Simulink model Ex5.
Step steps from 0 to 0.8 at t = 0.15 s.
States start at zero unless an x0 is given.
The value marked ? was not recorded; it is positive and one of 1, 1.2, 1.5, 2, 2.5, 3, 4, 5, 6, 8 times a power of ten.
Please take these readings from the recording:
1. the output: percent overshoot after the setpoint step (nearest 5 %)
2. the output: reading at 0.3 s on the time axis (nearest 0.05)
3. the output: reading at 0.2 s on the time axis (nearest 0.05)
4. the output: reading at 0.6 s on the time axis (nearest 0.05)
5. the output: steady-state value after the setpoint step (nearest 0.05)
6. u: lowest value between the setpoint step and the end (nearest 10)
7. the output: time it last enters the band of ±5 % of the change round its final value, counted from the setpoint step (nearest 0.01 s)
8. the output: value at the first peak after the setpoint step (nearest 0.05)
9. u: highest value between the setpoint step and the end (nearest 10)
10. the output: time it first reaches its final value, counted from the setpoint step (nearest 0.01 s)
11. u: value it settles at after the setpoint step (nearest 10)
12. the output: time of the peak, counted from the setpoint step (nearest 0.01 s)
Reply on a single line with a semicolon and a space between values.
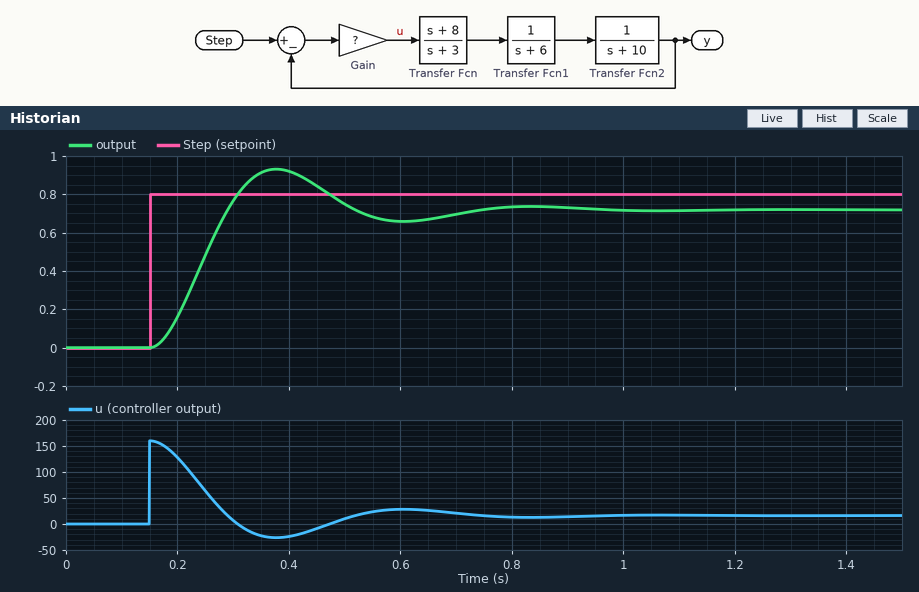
30 %; 0.75; 0.15; 0.65; 0.70; -30; 0.53 s; 0.95; 160; 0.14 s; 20; 0.23 s
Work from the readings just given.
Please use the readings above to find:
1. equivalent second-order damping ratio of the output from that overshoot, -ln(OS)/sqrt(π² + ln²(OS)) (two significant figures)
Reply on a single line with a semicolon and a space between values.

0.36
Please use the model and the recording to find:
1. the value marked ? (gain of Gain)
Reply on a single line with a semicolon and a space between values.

200
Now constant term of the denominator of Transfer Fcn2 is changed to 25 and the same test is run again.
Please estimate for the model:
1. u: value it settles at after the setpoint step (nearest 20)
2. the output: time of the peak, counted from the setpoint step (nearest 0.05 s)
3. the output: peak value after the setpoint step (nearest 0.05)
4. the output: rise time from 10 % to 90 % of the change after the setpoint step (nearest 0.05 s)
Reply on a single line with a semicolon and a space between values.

40; 0.30 s; 0.65; 0.15 s
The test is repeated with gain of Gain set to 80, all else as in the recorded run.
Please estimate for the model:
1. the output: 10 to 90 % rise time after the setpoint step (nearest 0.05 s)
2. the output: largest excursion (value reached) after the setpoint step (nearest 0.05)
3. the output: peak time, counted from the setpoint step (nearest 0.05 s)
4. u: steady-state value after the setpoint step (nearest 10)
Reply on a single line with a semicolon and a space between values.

0.15 s; 0.70; 0.35 s; 10
